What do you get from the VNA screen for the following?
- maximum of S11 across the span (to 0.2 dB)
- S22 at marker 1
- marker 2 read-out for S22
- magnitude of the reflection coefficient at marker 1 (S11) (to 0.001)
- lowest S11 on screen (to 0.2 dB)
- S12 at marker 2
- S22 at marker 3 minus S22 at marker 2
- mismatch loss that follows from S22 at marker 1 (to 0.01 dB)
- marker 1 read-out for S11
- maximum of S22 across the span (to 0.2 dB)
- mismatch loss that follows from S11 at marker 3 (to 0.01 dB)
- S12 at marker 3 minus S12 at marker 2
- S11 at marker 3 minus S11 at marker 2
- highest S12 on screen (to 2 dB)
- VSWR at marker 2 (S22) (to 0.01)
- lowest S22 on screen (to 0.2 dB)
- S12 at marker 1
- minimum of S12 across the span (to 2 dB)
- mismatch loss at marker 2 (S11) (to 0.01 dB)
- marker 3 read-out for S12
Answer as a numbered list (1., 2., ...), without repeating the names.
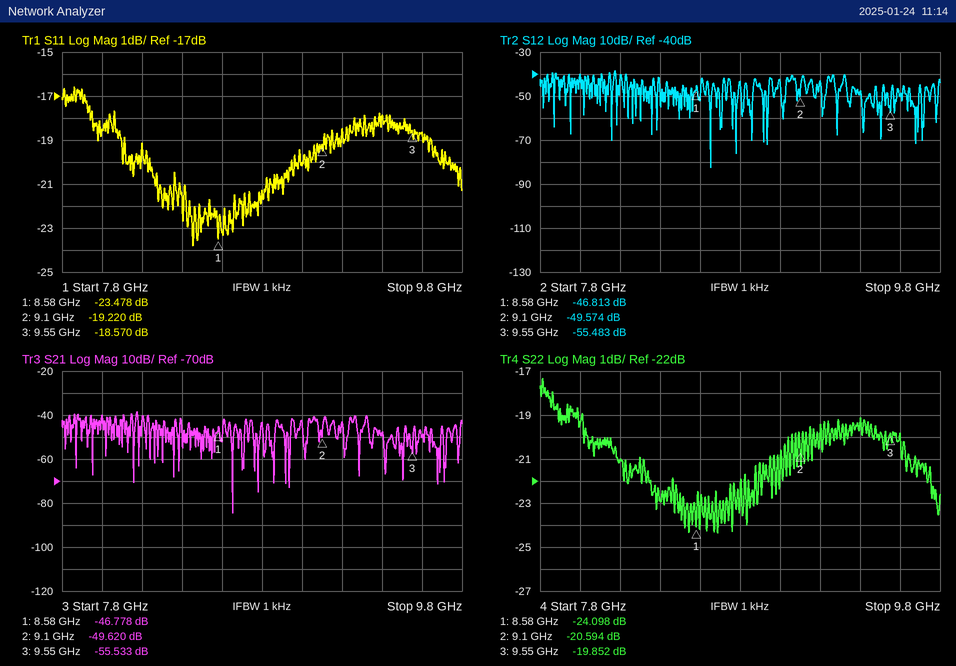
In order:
1. -16.6 dB
2. -24.098 dB
3. -20.594 dB
4. 0.067
5. -23.8 dB
6. -49.574 dB
7. 0.742 dB
8. 0.02 dB
9. -23.478 dB
10. -17.4 dB
11. 0.06 dB
12. -5.909 dB
13. 0.650 dB
14. -38 dB
15. 1.21
16. -24.4 dB
17. -46.813 dB
18. -82 dB
19. 0.05 dB
20. -55.483 dB
